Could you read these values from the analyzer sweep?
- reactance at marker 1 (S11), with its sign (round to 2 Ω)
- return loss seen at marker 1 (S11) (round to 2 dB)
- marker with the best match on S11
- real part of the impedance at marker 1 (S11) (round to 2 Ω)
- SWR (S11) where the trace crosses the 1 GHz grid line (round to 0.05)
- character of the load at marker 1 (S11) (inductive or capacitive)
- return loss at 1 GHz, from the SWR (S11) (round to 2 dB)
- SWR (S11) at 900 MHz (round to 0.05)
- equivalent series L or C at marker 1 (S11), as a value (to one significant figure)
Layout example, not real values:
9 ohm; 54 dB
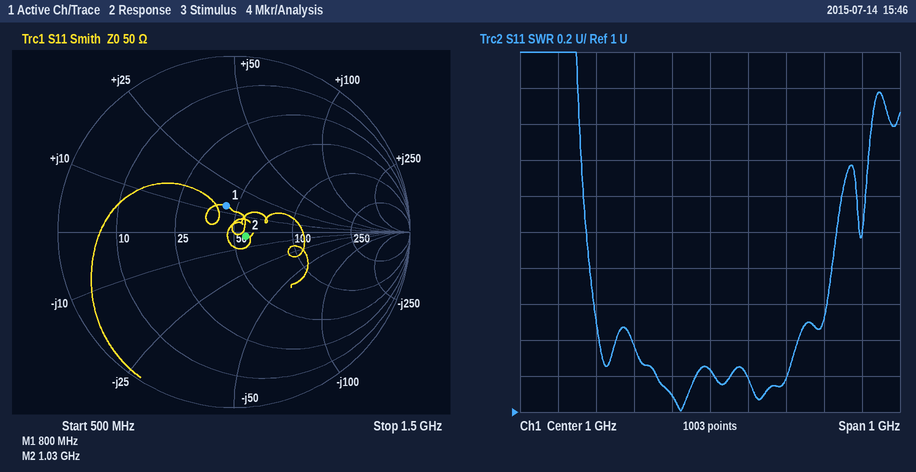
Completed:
+14 Ω; 16 dB; marker 2; 44 Ω; 1.25; inductive; 20 dB; 1.10; 3 nH
